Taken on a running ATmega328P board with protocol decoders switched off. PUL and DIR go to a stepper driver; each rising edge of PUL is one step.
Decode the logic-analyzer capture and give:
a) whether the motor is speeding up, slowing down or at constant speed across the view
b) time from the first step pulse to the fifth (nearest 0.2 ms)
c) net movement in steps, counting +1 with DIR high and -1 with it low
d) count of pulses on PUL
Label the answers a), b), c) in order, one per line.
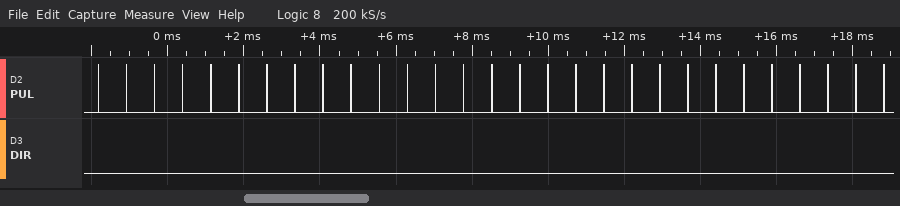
a) constant speed
b) 3.0 ms
c) -29
d) 29
